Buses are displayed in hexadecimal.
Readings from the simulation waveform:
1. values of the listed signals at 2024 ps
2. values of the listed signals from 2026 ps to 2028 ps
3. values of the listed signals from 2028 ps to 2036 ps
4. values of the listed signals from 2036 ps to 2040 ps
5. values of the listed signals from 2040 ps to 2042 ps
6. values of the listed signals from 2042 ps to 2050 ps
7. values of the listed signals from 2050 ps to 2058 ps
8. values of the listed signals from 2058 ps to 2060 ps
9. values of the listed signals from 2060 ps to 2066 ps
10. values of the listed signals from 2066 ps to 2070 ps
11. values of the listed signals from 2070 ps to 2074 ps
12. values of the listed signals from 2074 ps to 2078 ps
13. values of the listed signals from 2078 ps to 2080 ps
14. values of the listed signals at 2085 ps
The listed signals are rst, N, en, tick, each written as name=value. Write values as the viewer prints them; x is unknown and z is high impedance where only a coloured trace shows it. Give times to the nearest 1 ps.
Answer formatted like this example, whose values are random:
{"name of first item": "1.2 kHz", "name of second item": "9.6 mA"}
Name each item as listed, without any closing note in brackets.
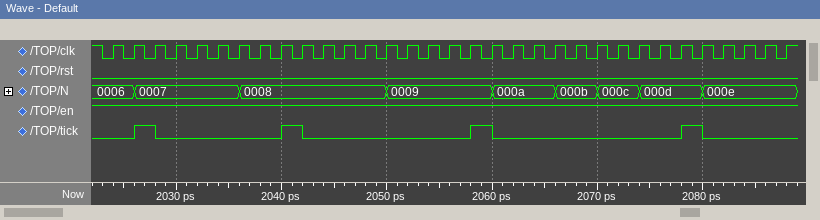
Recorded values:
{"values of the listed signals at 2024 ps": "rst=0, N=0006, en=1, tick=0", "values of the listed signals from 2026 ps to 2028 ps": "rst=0, N=0007, en=1, tick=1", "values of the listed signals from 2028 ps to 2036 ps": "rst=0, N=0007, en=1, tick=0", "values of the listed signals from 2036 ps to 2040 ps": "rst=0, N=0008, en=1, tick=0", "values of the listed signals from 2040 ps to 2042 ps": "rst=0, N=0008, en=1, tick=1", "values of the listed signals from 2042 ps to 2050 ps": "rst=0, N=0008, en=1, tick=0", "values of the listed signals from 2050 ps to 2058 ps": "rst=0, N=0009, en=1, tick=0", "values of the listed signals from 2058 ps to 2060 ps": "rst=0, N=0009, en=1, tick=1", "values of the listed signals from 2060 ps to 2066 ps": "rst=0, N=000a, en=1, tick=0", "values of the listed signals from 2066 ps to 2070 ps": "rst=0, N=000b, en=1, tick=0", "values of the listed signals from 2070 ps to 2074 ps": "rst=0, N=000c, en=1, tick=0", "values of the listed signals from 2074 ps to 2078 ps": "rst=0, N=000d, en=1, tick=0", "values of the listed signals from 2078 ps to 2080 ps": "rst=0, N=000d, en=1, tick=1", "values of the listed signals at 2085 ps": "rst=0, N=000e, en=1, tick=0"}
